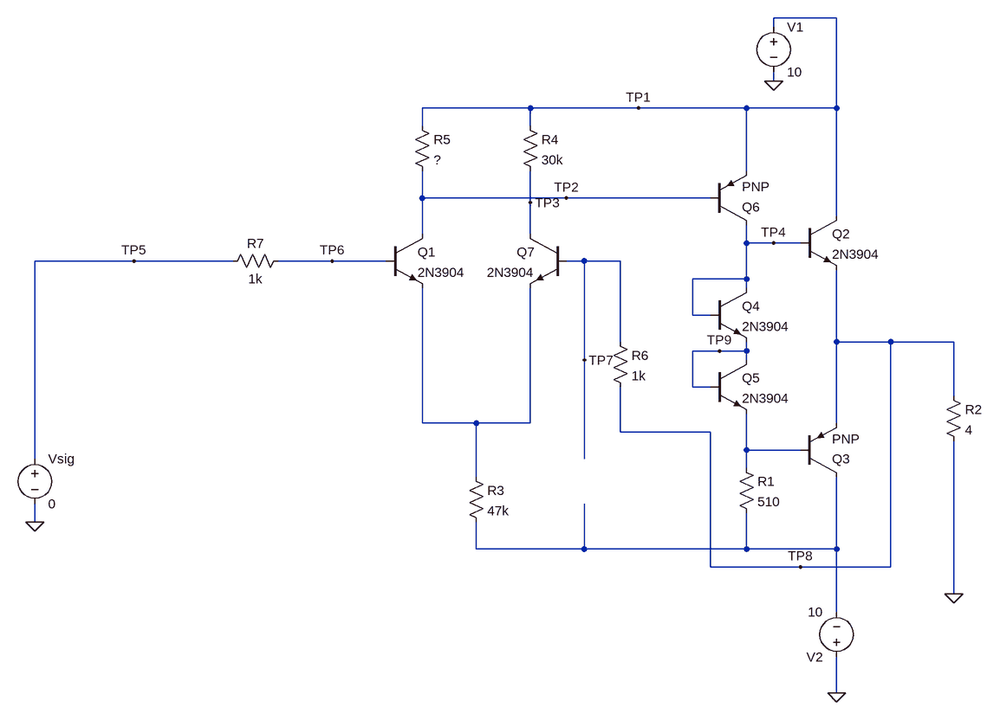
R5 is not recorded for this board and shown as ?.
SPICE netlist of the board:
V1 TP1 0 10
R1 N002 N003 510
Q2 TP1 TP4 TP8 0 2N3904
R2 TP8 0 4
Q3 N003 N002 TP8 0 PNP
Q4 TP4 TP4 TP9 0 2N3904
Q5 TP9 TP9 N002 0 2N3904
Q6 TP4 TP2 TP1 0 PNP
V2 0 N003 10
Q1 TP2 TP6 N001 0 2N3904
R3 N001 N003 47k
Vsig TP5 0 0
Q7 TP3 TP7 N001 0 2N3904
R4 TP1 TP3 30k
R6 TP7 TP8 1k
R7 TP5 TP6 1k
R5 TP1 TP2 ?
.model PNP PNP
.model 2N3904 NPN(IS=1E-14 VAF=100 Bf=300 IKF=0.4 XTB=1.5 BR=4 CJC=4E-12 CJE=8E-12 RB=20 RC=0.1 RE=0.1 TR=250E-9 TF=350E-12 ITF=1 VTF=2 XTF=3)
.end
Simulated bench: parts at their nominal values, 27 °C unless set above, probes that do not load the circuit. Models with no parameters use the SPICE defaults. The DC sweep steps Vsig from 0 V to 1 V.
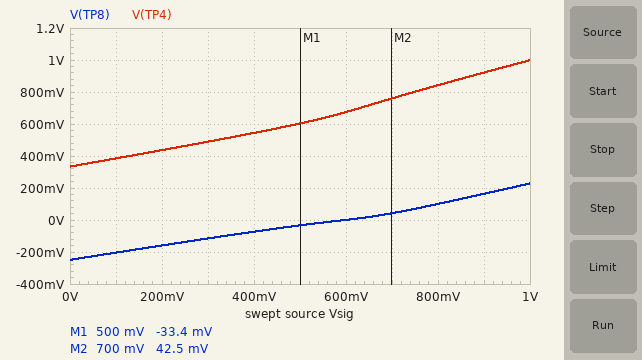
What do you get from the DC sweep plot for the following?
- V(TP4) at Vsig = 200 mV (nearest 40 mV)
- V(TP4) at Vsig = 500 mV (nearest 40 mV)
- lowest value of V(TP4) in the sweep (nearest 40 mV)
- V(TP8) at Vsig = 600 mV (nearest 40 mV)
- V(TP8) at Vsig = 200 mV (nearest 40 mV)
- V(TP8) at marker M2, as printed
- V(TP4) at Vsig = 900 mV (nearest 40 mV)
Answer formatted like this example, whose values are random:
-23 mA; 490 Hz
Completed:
440 mV; 600 mV; 320 mV; 0 V; -160 mV; 42.5 mV; 920 mV
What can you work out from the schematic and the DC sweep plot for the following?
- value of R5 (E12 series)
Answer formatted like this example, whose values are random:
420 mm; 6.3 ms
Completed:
27 kΩ
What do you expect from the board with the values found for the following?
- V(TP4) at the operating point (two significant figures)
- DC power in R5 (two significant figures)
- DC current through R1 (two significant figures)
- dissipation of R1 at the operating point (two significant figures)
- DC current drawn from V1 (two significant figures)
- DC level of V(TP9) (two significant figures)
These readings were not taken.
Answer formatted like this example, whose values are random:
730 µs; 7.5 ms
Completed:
330 mV; 27 µW; 17 mA; 150 mW; 17 mA; -400 mV
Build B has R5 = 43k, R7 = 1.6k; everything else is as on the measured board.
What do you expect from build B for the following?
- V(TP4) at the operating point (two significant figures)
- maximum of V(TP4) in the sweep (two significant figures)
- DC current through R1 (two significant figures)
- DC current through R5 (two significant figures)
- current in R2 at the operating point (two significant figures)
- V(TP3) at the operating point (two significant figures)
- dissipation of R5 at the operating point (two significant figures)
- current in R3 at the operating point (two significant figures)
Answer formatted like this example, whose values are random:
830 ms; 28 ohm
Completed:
510 mV; 1.4 V; 18 mA; 20 µA; 25 mA; 9.9 V; 17 µW; 200 µA
